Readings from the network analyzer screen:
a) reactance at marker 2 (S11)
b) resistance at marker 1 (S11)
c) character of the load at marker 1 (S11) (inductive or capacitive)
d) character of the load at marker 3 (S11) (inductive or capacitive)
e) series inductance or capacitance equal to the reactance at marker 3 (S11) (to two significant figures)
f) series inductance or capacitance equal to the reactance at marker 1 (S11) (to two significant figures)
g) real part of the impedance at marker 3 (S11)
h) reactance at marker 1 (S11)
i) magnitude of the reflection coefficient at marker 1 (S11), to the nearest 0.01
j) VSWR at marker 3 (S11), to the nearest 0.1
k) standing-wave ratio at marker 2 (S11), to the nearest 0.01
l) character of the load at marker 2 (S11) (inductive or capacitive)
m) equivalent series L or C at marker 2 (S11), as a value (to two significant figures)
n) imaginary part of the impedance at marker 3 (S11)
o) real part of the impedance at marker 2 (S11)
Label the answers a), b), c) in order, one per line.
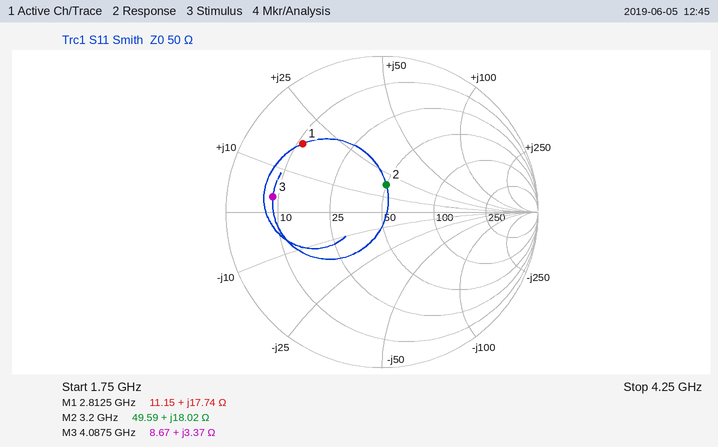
a) +18.02 Ω
b) 11.15 Ω
c) inductive
d) inductive
e) 130 pH
f) 1.0 nH
g) 8.67 Ω
h) +17.74 Ω
i) 0.67
j) 5.8
k) 1.43
l) inductive
m) 900 pH
n) +3.37 Ω
o) 49.59 Ω
